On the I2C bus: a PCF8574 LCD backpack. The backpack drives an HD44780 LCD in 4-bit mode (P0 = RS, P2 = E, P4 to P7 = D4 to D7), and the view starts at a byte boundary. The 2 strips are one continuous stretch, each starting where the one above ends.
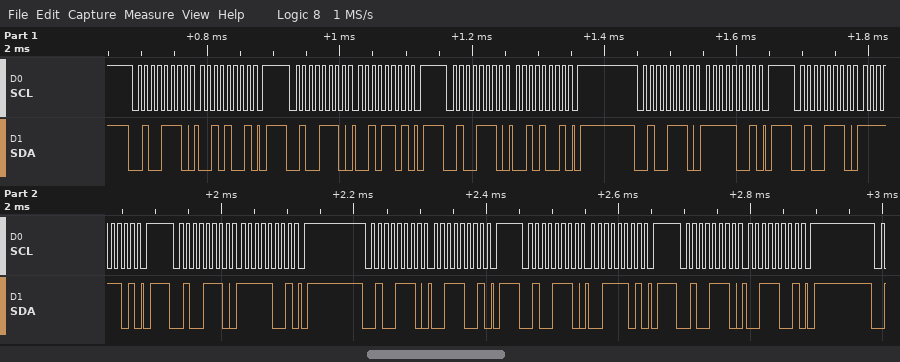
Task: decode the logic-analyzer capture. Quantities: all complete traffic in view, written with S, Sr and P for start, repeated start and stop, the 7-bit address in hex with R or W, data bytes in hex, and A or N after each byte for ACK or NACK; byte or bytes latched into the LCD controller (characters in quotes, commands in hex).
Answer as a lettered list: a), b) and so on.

a) S 27W A 29 A P S 27W A 2D A P S 27W A 29 A P S 27W A F9 A P S 27W A FD A P S 27W A F9 A P S 27W A 39 A P S 27W A 3D A P S 27W A 39 A P
b) '/'
